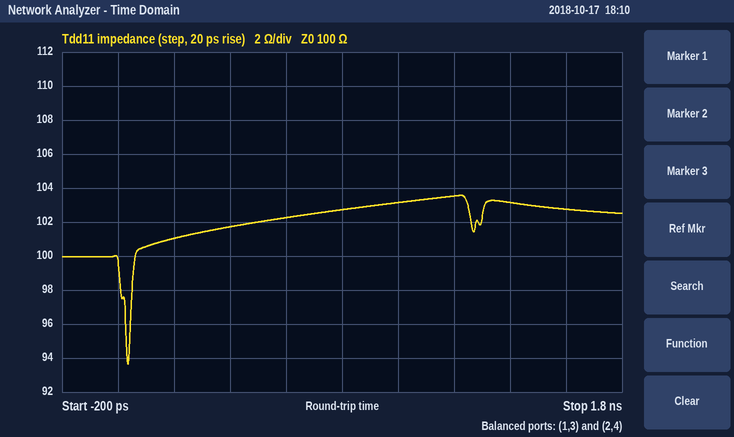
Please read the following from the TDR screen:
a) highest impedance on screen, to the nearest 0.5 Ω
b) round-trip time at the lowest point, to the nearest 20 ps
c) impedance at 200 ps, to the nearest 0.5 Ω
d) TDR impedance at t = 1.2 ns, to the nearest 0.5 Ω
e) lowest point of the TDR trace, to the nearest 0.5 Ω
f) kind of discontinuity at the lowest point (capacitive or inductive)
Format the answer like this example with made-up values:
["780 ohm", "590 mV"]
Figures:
["103.5 Ω", "40 ps", "101.0 Ω", "103.5 Ω", "93.5 Ω", "capacitive"]
